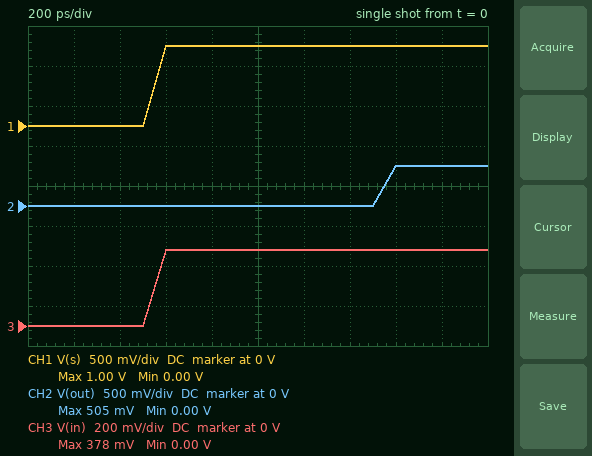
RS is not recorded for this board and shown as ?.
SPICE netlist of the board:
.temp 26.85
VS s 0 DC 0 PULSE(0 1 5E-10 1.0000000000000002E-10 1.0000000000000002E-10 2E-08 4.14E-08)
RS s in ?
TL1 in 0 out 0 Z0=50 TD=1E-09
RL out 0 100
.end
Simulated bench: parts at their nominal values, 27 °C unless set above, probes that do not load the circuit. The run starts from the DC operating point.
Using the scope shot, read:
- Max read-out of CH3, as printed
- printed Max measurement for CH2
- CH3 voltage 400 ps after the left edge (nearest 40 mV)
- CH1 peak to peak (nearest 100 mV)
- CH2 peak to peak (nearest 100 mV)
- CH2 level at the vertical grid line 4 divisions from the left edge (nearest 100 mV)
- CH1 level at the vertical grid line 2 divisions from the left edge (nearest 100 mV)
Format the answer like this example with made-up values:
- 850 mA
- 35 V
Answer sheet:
- 378 mV
- 505 mV
- 0 V
- 1.0 V
- 500 mV
- 0 V
- 0 V
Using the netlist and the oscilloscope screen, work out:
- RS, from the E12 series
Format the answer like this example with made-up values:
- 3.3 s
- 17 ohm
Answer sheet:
- 82 Ω
